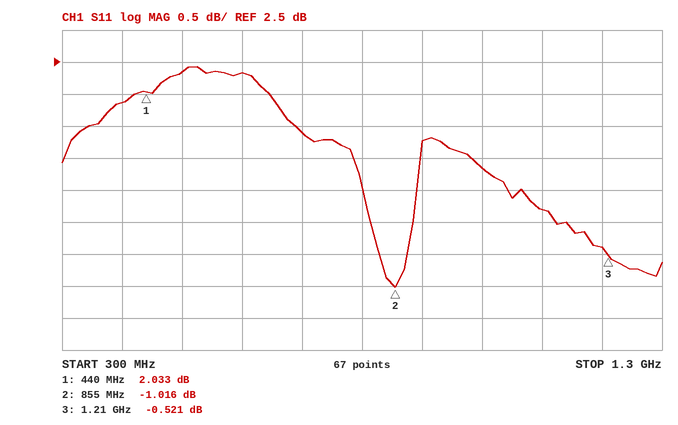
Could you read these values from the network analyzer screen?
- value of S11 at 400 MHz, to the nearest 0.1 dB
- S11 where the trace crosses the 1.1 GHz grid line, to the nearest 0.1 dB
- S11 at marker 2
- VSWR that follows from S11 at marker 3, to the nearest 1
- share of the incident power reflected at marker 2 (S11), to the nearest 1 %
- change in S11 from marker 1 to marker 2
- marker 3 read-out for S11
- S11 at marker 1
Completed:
1.9 dB
0.2 dB
-1.016 dB
33
79 %
-3.049 dB
-0.521 dB
2.033 dB
